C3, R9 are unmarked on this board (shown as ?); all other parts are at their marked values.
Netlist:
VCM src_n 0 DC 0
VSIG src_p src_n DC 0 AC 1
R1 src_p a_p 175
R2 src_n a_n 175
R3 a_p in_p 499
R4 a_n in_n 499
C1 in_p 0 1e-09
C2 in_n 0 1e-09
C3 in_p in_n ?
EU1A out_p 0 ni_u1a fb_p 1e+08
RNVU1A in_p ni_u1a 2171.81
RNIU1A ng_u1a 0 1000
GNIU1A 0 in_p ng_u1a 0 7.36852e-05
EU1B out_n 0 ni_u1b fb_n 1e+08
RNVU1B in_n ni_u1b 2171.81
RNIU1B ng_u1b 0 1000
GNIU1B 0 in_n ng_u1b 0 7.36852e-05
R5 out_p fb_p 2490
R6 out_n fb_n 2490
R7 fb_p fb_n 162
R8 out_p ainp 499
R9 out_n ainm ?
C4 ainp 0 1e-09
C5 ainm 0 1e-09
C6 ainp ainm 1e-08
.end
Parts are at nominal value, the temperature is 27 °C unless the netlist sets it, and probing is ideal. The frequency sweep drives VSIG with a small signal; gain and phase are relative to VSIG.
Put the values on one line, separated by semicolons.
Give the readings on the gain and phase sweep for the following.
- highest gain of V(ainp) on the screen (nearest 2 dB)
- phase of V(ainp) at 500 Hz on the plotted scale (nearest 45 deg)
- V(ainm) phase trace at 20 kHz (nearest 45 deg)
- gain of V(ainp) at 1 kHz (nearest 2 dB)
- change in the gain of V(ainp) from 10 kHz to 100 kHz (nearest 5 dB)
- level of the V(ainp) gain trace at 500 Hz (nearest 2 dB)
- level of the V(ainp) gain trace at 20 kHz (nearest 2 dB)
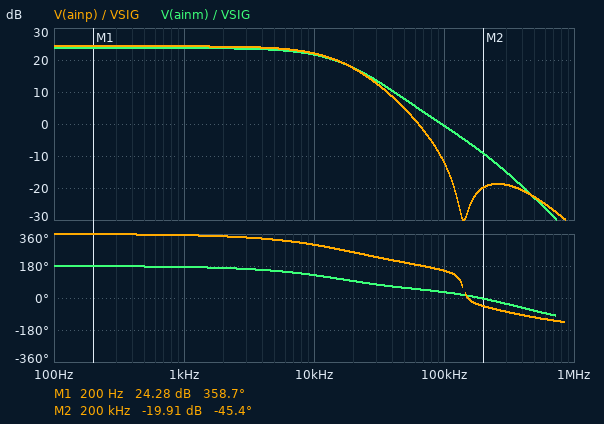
24 dB; 360 deg; 90 deg; 24 dB; -35 dB; 24 dB; 18 dB
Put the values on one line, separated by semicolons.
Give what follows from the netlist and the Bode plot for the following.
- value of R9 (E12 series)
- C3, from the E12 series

330 Ω; 5.6 nF
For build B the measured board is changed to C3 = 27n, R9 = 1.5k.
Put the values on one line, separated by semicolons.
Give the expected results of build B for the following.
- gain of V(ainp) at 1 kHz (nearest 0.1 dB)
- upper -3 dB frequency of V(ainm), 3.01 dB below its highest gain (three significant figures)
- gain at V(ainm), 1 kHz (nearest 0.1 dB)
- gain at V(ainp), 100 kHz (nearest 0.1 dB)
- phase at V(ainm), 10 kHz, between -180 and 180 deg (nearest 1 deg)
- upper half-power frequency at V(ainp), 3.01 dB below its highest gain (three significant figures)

24.0 dB; 3.75 kHz; 23.5 dB; -4.0 dB; 23 deg; 3.64 kHz
